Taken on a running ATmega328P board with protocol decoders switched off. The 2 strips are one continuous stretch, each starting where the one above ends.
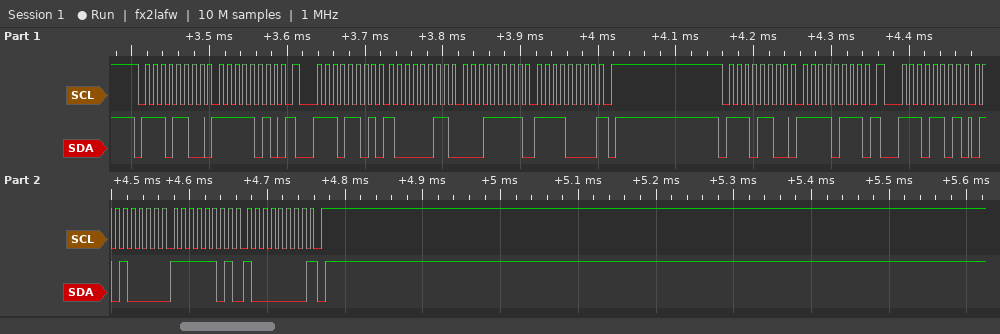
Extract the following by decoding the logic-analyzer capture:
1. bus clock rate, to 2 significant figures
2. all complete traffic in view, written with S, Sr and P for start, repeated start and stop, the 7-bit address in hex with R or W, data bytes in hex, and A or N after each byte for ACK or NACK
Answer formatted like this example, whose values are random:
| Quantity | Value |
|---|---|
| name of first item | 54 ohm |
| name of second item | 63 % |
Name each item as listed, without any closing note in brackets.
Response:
| Quantity | Value |
|---|---|
| bus clock rate, to 2 significant figures | 100 kHz |
| all complete traffic in view, written with S, Sr and P for start, repeated start and stop, the 7-bit address in hex with R or W, data bytes in hex, and A or N after each byte for ACK or NACK | S 76W A FA A Sr 76R A 83 A 1F A F0 N P S 76W A F7 A Sr 76R A 50 A FD A 80 N P |
